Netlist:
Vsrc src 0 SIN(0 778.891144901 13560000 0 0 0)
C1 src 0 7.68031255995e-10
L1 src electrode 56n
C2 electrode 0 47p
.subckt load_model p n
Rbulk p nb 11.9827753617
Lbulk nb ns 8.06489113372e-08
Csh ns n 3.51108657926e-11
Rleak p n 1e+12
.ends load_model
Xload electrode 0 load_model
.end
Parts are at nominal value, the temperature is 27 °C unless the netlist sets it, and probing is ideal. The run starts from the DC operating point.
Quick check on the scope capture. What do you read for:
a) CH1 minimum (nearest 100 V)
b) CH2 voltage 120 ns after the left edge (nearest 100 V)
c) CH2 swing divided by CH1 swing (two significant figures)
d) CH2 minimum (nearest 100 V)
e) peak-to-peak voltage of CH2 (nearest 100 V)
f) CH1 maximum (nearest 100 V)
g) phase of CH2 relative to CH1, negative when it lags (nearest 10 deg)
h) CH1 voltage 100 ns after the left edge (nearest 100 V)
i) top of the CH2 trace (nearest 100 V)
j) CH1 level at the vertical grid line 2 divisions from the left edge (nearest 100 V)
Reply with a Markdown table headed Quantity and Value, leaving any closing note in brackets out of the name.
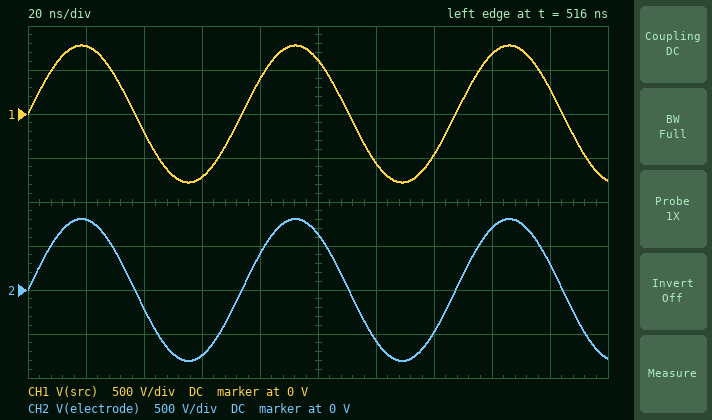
| Quantity | Value |
|---|---|
| CH1 minimum | -800 V |
| CH2 voltage 120 ns after the left edge | -600 V |
| CH2 swing divided by CH1 swing | 1.0 |
| CH2 minimum | -800 V |
| peak-to-peak voltage of CH2 | 1.6 kV |
| CH1 maximum | 800 V |
| phase of CH2 relative to CH1, negative when it lags | 0 deg |
| CH1 voltage 100 ns after the left edge | 600 V |
| top of the CH2 trace | 800 V |
| CH1 level at the vertical grid line 2 divisions from the left edge | -200 V |
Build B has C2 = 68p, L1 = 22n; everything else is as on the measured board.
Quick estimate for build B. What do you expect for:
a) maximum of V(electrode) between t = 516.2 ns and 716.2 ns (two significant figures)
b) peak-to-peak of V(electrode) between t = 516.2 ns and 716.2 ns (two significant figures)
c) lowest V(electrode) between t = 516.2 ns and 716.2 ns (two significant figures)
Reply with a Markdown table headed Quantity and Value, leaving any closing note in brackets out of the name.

| Quantity | Value |
|---|---|
| maximum of V(electrode) between t = 516.2 ns and 716.2 ns | 790 V |
| peak-to-peak of V(electrode) between t = 516.2 ns and 716.2 ns | 1.6 kV |
| lowest V(electrode) between t = 516.2 ns and 716.2 ns | -790 V |
